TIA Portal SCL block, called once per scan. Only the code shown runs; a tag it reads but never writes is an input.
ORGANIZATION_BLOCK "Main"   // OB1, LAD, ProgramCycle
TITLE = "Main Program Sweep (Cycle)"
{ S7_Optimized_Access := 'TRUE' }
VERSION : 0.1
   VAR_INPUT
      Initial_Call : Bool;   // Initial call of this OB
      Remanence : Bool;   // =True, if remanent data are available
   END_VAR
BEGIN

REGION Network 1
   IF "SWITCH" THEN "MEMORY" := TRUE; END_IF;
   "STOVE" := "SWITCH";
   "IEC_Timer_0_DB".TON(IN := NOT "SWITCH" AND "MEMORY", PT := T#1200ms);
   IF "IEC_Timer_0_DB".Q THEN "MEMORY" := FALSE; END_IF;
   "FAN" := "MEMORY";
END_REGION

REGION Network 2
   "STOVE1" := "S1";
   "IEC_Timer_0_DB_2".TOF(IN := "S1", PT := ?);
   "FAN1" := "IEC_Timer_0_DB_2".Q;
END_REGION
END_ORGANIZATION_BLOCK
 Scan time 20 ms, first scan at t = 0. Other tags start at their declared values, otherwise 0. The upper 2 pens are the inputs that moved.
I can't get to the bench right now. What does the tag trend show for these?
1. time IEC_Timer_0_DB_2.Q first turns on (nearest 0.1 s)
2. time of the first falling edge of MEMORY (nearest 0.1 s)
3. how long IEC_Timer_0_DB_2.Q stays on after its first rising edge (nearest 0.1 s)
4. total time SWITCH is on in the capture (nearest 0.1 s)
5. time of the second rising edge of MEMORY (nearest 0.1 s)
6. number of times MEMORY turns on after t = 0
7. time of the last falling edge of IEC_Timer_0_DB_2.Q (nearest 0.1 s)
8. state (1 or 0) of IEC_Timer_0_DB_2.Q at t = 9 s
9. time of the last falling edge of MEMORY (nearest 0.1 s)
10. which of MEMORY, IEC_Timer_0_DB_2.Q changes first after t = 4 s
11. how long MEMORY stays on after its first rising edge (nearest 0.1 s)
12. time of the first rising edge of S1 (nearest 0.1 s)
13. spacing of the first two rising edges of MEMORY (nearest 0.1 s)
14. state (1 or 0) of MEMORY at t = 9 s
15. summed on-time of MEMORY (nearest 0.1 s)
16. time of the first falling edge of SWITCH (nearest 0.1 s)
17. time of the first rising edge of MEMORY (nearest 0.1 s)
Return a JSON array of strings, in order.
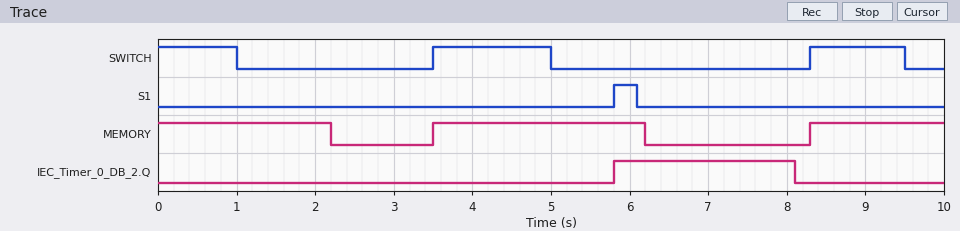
["5.8 s", "2.2 s", "2.3 s", "3.7 s", "8.3 s", "2", "8.1 s", "0", "6.2 s", "IEC_Timer_0_DB_2.Q", "2.7 s", "5.8 s", "4.8 s", "1", "6.6 s", "1.0 s", "3.5 s"]
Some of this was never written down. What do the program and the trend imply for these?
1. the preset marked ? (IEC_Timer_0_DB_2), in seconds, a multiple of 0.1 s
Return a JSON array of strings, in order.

["2.0 s"]
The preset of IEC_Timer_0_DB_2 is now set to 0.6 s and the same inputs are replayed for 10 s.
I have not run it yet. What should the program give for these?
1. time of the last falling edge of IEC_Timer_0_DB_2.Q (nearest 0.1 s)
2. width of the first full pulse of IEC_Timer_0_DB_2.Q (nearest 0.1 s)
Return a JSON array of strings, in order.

["6.7 s", "0.9 s"]
